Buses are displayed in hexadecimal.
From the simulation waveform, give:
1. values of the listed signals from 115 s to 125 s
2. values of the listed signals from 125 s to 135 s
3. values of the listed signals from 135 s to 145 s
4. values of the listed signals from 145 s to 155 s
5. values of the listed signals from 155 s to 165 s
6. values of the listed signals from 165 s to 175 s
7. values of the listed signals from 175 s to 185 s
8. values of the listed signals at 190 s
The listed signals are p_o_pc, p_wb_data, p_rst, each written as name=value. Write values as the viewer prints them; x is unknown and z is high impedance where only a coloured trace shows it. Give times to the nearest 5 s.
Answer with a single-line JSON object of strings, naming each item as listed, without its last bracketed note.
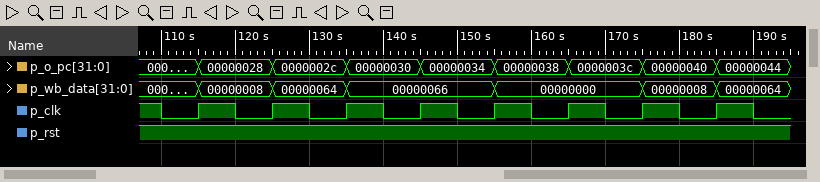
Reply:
{"values of the listed signals from 115 s to 125 s": "p_o_pc=00000028, p_wb_data=00000008, p_rst=1", "values of the listed signals from 125 s to 135 s": "p_o_pc=0000002c, p_wb_data=00000064, p_rst=1", "values of the listed signals from 135 s to 145 s": "p_o_pc=00000030, p_wb_data=00000066, p_rst=1", "values of the listed signals from 145 s to 155 s": "p_o_pc=00000034, p_wb_data=00000066, p_rst=1", "values of the listed signals from 155 s to 165 s": "p_o_pc=00000038, p_wb_data=00000000, p_rst=1", "values of the listed signals from 165 s to 175 s": "p_o_pc=0000003c, p_wb_data=00000000, p_rst=1", "values of the listed signals from 175 s to 185 s": "p_o_pc=00000040, p_wb_data=00000008, p_rst=1", "values of the listed signals at 190 s": "p_o_pc=00000044, p_wb_data=00000064, p_rst=1"}
